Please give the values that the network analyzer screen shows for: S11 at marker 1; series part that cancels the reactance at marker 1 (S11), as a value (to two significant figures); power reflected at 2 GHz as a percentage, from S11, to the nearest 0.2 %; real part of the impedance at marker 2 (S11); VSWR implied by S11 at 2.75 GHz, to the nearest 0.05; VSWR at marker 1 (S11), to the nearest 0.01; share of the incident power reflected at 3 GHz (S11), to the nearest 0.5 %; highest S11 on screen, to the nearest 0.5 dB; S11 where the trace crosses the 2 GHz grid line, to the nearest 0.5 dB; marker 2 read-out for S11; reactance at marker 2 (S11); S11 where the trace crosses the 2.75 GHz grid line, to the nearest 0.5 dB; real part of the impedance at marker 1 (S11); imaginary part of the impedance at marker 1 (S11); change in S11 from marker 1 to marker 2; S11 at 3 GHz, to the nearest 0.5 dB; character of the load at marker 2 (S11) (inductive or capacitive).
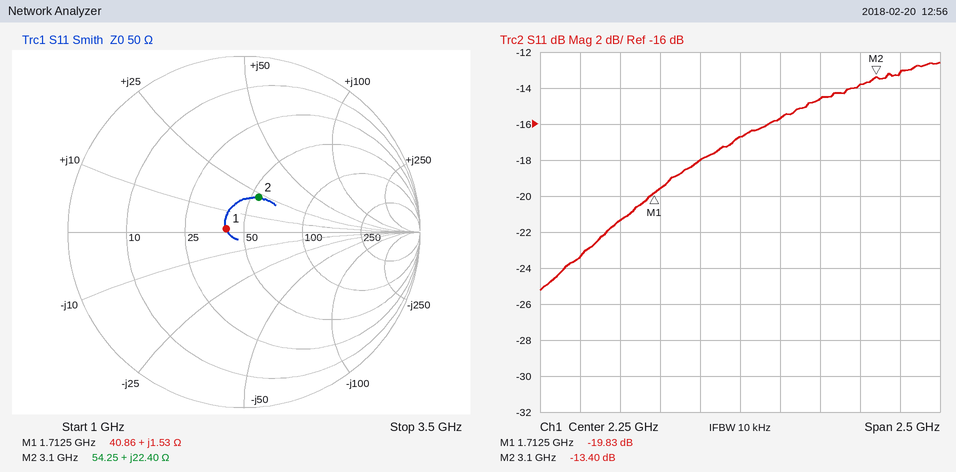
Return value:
-19.83 dB
61 pF
1.6 %
54.25 Ω
1.45
1.23
4.0 %
-12.5 dB
-18.0 dB
-13.40 dB
+22.40 Ω
-14.5 dB
40.86 Ω
+1.53 Ω
6.43 dB
-14.0 dB
inductive
